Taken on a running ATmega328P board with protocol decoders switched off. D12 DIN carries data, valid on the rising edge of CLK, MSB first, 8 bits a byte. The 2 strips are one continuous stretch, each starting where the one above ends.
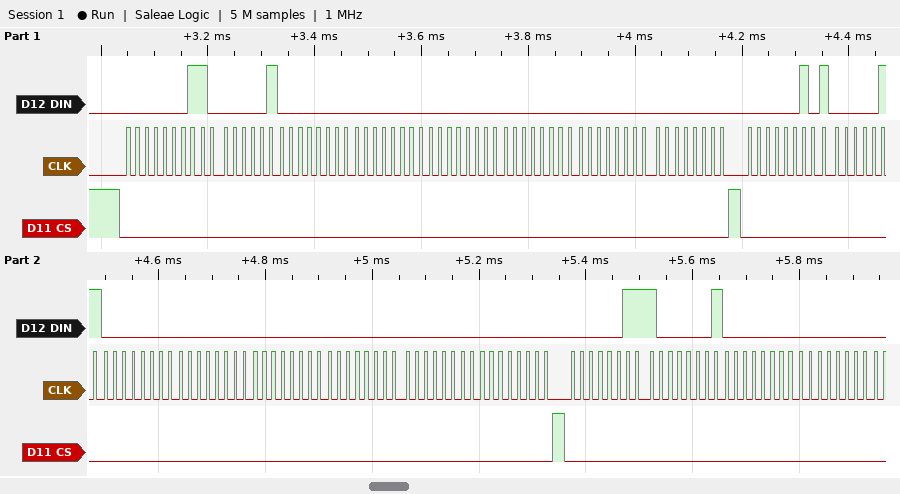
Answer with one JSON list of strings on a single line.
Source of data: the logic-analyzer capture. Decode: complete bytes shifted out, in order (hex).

["01 81 00 00 00 00 00 00 02 83 00 00 00 00 00 00 03 81 00 00"]
